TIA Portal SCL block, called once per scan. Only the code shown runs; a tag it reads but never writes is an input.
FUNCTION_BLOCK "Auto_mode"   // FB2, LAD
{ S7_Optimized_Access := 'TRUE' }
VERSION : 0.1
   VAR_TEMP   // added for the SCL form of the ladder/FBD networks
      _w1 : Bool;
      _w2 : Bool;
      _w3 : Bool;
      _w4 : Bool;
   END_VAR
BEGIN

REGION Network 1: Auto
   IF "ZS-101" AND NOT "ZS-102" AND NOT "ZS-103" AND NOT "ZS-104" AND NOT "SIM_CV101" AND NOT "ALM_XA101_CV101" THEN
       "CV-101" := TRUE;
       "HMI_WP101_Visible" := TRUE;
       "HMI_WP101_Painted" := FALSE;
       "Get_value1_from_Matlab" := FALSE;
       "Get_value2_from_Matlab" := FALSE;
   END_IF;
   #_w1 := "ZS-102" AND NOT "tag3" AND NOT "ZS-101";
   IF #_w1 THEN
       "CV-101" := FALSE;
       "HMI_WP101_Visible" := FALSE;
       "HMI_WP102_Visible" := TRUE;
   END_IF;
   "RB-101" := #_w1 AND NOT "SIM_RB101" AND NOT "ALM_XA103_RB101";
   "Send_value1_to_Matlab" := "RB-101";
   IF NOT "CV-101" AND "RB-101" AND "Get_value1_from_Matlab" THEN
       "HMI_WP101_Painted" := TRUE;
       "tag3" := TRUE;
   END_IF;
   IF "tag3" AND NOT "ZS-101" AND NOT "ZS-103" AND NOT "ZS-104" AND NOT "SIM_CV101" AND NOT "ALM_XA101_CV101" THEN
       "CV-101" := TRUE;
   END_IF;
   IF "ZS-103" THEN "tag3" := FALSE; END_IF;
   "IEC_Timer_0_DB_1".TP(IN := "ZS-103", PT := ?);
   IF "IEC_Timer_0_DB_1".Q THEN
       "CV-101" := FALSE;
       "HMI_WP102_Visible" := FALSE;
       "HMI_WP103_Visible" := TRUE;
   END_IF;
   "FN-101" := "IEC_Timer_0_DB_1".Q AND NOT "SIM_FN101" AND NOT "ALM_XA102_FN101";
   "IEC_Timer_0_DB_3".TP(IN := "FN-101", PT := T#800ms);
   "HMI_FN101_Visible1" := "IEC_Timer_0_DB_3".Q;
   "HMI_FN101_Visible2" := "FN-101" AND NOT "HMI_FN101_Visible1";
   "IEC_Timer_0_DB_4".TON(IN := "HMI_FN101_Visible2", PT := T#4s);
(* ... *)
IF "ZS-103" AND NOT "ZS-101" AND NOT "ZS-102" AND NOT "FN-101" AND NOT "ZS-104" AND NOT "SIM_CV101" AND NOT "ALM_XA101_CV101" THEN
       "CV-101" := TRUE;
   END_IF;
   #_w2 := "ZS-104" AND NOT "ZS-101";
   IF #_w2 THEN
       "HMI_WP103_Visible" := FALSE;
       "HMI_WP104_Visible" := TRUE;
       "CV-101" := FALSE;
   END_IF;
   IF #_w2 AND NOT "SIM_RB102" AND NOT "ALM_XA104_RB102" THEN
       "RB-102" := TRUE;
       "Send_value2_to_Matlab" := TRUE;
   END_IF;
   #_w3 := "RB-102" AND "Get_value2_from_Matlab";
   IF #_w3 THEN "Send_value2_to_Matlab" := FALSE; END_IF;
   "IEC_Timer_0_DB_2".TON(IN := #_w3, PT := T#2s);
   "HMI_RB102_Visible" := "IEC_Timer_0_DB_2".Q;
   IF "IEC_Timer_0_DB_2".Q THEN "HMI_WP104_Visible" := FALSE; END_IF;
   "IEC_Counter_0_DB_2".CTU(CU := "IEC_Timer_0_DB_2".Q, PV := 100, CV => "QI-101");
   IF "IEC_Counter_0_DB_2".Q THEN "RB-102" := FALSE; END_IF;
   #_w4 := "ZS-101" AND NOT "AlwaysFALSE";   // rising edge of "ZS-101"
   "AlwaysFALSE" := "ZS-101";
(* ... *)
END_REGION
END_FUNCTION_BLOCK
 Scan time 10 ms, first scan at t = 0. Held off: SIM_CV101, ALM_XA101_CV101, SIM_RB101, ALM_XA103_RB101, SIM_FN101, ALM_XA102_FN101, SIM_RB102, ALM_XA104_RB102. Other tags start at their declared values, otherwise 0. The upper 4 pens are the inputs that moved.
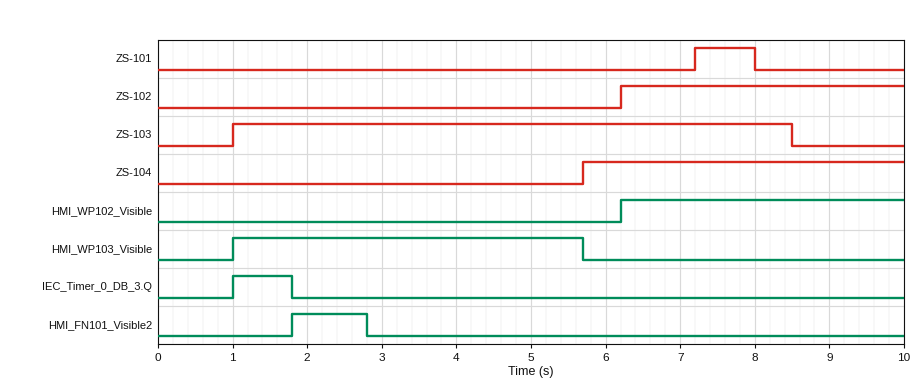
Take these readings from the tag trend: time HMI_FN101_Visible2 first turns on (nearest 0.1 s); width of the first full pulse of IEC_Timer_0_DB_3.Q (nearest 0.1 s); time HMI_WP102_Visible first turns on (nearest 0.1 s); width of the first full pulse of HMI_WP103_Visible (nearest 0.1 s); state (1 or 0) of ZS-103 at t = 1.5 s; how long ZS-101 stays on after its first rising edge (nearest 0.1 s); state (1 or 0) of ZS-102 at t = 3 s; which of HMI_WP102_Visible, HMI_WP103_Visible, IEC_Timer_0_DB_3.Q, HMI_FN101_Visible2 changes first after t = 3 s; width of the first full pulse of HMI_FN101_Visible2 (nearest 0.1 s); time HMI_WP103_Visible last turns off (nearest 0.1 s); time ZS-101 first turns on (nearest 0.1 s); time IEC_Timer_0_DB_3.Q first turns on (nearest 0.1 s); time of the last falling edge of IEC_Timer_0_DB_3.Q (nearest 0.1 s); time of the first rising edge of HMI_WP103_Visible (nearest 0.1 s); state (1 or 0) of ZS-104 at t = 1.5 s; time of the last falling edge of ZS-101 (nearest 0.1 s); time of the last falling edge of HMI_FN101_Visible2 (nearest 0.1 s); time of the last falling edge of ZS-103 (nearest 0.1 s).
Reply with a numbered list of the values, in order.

1. 1.8 s
2. 0.8 s
3. 6.2 s
4. 4.7 s
5. 1
6. 0.8 s
7. 0
8. HMI_WP103_Visible
9. 1.0 s
10. 5.7 s
11. 7.2 s
12. 1.0 s
13. 1.8 s
14. 1.0 s
15. 0
16. 8.0 s
17. 2.8 s
18. 8.5 s
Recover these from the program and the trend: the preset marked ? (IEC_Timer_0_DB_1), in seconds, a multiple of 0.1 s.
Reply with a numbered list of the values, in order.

1. 1.8 s
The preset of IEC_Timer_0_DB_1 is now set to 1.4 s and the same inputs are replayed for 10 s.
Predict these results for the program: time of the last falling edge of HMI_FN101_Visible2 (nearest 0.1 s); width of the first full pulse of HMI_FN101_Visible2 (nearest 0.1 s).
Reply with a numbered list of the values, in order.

1. 2.4 s
2. 0.6 s
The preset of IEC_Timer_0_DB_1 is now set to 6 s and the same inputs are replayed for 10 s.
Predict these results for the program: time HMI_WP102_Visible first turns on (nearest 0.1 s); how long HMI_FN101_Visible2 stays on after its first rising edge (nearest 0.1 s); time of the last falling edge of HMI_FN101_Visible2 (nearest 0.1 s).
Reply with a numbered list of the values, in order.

1. 7.0 s
2. 5.2 s
3. 7.0 s
